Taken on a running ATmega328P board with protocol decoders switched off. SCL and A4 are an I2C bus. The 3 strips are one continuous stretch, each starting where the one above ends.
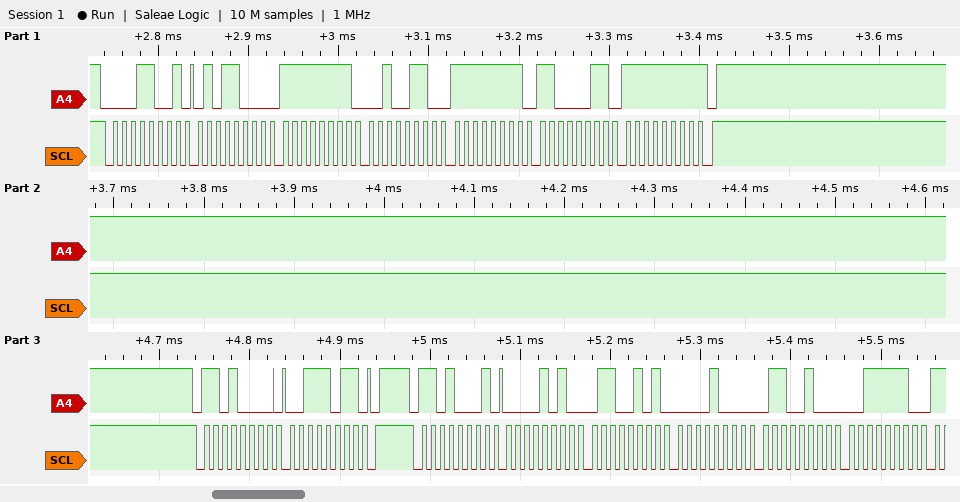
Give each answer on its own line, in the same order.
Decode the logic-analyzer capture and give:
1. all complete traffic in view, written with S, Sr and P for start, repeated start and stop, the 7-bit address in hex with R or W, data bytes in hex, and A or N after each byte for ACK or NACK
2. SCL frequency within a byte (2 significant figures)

S 0CR A 58 A FF A 26 A FF A C3 A FF N P S 68W A 3B A P S 68R A 0A A 65 A 08 A 64 A 3E A
100 kHz
